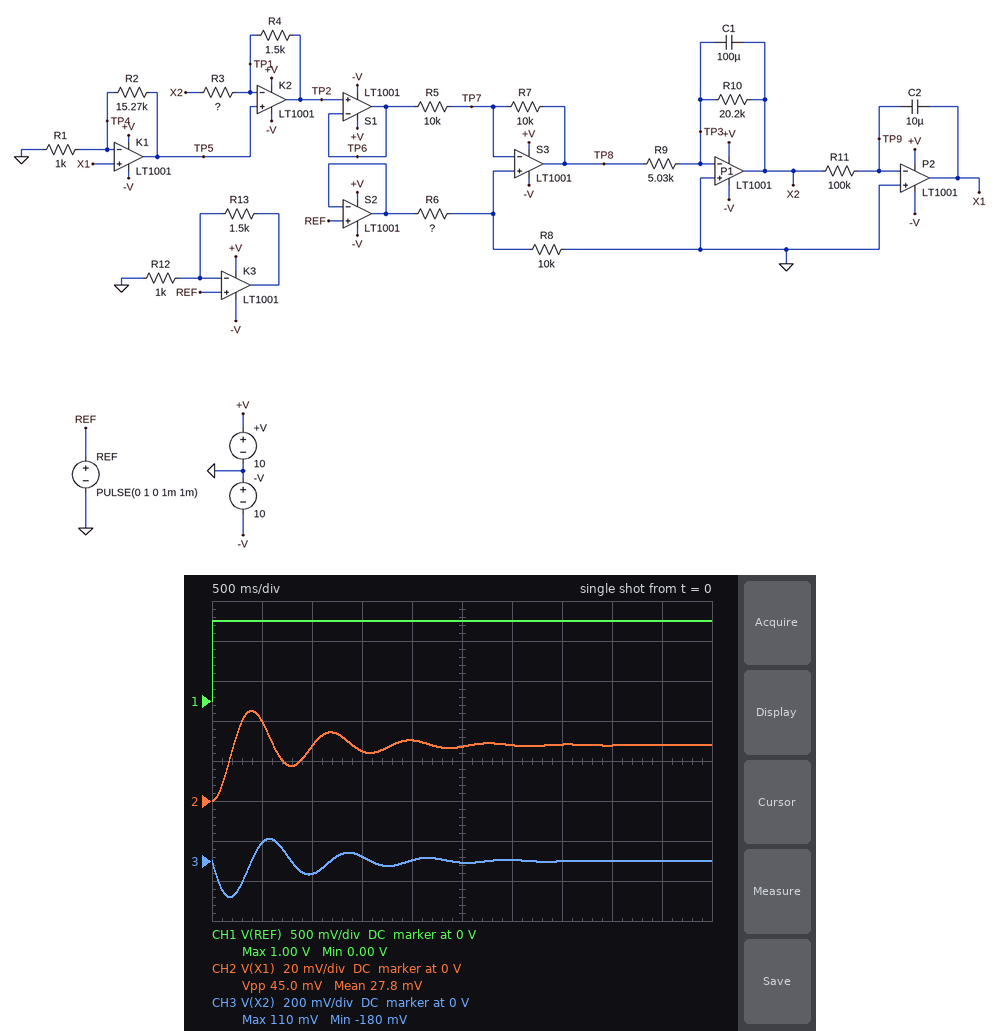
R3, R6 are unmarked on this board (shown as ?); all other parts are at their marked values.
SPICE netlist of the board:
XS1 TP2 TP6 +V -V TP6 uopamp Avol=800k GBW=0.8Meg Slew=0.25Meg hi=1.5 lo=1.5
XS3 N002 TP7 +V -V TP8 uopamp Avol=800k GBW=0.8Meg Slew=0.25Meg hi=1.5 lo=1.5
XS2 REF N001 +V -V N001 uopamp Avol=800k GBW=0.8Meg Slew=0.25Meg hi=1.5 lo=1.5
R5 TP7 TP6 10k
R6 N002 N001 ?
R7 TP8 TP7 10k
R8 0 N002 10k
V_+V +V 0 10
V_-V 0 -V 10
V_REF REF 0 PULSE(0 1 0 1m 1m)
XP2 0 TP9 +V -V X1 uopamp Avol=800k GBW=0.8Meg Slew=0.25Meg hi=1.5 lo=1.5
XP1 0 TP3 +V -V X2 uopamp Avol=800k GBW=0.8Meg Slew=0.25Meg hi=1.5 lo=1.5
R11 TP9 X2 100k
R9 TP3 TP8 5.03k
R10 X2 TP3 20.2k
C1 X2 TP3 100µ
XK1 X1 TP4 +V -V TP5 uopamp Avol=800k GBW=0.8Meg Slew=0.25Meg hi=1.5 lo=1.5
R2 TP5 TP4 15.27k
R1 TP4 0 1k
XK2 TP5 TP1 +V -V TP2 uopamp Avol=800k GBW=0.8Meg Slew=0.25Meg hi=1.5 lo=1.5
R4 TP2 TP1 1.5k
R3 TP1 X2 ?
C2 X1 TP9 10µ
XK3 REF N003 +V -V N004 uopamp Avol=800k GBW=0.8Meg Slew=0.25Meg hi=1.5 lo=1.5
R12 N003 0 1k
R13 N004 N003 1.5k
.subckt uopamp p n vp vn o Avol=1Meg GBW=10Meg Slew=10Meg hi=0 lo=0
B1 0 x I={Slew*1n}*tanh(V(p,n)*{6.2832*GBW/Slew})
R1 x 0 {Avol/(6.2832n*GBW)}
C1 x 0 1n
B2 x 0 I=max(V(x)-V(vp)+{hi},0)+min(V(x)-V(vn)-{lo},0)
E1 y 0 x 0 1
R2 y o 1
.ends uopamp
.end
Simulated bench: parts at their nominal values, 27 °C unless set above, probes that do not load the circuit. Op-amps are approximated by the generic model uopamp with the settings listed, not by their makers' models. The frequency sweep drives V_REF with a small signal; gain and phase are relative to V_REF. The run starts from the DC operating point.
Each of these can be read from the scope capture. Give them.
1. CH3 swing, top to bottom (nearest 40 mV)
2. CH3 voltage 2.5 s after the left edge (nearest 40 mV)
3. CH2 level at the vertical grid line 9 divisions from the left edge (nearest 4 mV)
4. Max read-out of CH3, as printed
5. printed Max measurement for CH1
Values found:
280 mV
0 V
28 mV
110 mV
1.00 V
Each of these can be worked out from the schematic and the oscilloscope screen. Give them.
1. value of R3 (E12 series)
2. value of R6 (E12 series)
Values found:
1.5 kΩ
12 kΩ
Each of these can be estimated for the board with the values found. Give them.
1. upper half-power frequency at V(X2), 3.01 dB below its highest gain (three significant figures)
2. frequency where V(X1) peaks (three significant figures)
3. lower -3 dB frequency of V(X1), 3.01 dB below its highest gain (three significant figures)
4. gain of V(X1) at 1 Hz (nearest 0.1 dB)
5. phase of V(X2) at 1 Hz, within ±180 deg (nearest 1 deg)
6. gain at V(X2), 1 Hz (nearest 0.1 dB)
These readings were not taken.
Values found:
1.49 Hz
1.25 Hz
1.03 Hz
-24.3 dB
-122 deg
-8.3 dB
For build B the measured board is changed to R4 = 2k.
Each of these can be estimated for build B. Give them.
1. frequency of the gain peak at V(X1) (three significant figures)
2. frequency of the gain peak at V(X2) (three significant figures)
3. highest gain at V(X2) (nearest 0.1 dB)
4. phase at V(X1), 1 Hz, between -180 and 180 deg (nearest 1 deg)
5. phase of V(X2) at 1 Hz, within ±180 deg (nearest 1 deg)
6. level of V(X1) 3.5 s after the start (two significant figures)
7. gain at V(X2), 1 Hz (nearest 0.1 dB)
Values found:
1.34 Hz
1.38 Hz
-4.8 dB
-29 deg
-119 deg
24 mV
-11.2 dB
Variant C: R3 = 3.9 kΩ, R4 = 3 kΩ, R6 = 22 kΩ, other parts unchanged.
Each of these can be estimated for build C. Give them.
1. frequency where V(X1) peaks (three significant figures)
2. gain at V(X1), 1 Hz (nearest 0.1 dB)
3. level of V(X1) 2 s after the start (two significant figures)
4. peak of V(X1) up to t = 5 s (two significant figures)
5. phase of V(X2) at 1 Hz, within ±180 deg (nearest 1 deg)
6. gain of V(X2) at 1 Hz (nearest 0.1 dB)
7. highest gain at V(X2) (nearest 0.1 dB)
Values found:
1.18 Hz
-24.9 dB
24 mV
36 mV
-126 deg
-8.9 dB
-4.2 dB
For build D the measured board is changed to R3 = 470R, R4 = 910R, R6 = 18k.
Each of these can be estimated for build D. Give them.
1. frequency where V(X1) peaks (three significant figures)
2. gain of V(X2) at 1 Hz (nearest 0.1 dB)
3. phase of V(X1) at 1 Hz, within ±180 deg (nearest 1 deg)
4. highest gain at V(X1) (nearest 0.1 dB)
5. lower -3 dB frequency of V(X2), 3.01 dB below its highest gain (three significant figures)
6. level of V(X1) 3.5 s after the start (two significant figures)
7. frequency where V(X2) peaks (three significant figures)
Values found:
1.47 Hz
-16.8 dB
-26 deg
-29.3 dB
1.24 Hz
15 mV
1.55 Hz
